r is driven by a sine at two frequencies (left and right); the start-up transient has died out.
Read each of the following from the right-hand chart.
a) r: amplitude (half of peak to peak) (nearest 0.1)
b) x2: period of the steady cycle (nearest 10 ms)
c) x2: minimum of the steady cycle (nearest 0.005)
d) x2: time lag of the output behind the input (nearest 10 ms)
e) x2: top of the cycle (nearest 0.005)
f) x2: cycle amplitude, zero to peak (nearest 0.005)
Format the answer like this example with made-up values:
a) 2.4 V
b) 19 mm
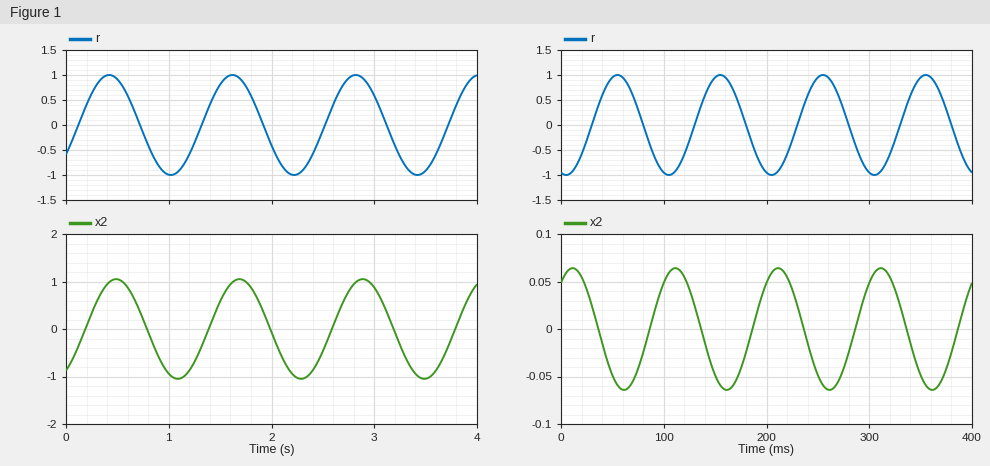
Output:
a) 1.0
b) 100 ms
c) -0.065
d) 60 ms
e) 0.065
f) 0.065
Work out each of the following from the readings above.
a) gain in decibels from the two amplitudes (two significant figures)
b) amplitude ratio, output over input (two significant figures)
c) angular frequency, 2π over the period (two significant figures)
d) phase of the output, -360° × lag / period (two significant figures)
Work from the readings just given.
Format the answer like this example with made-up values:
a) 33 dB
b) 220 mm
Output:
a) -24 dB
b) 0.065
c) 0.063 rad/ms
d) -220°
